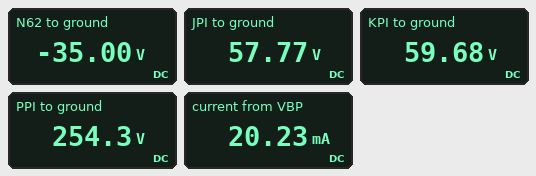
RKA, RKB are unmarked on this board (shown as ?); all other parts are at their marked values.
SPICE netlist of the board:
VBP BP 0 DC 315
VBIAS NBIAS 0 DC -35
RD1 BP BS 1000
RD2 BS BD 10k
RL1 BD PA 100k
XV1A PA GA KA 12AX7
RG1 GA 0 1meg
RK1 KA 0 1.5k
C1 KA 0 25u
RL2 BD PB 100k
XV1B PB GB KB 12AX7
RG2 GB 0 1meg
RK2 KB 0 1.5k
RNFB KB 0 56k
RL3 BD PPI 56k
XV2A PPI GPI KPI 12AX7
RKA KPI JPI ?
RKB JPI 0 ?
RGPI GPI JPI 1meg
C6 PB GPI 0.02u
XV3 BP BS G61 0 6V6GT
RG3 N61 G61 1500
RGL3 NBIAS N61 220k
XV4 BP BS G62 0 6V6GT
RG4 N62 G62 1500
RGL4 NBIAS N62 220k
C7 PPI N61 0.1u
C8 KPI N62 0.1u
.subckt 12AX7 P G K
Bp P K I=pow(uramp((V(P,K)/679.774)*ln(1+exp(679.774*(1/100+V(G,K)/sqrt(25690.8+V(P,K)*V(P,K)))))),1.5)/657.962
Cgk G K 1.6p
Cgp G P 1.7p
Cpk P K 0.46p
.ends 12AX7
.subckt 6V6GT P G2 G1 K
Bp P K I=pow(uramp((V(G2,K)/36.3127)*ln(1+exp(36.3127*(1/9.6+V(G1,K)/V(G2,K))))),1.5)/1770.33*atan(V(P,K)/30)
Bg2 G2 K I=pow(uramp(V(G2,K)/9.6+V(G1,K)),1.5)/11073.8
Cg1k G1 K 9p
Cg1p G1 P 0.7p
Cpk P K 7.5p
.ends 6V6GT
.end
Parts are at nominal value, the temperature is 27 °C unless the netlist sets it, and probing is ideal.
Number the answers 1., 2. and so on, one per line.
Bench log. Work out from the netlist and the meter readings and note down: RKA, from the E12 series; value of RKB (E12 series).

1. 3.3 kΩ
2. 100 kΩ
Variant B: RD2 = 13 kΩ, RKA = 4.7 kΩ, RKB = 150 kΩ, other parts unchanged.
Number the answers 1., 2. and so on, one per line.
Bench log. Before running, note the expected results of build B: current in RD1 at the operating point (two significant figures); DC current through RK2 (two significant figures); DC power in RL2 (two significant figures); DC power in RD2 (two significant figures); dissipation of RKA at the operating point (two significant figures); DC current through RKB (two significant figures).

1. 2.4 mA
2. 960 µA
3. 97 mW
4. 74 mW
5. 870 µW
6. 430 µA
